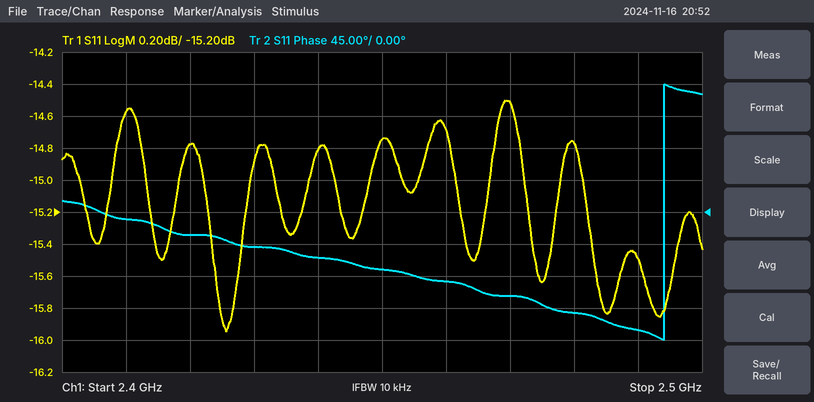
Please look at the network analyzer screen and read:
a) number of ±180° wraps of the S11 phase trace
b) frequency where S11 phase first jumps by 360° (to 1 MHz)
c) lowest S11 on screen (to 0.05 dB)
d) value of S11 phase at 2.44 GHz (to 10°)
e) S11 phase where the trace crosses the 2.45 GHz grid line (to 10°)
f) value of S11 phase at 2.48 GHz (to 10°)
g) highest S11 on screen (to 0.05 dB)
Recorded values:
1
2.494 GHz
-15.95 dB
-60°
-80°
-140°
-14.50 dB
